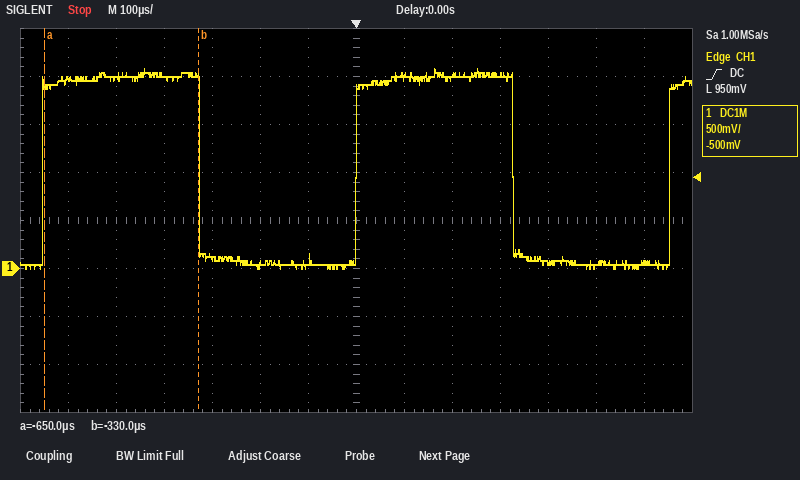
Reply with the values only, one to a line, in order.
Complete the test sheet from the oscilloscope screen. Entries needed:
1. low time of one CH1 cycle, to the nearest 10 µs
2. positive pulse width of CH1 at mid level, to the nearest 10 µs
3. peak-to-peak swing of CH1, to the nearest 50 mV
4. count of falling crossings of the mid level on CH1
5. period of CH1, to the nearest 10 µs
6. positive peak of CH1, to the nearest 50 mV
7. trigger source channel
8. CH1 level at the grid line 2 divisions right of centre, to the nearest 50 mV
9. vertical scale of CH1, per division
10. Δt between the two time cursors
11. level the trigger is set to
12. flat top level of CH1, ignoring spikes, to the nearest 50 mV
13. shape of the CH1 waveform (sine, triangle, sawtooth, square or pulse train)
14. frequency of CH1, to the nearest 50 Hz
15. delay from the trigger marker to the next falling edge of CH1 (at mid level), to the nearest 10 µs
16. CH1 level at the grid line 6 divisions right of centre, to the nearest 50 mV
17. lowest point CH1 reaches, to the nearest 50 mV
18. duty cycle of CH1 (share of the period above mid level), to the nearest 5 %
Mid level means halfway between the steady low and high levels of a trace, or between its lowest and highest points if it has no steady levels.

330 µs
330 µs
2.10 V
2
650 µs
2.10 V
CH1
2.00 V
500 mV
320 µs
950 mV
2.00 V
square
1.55 kHz
330 µs
50 mV
0 mV
50 %
